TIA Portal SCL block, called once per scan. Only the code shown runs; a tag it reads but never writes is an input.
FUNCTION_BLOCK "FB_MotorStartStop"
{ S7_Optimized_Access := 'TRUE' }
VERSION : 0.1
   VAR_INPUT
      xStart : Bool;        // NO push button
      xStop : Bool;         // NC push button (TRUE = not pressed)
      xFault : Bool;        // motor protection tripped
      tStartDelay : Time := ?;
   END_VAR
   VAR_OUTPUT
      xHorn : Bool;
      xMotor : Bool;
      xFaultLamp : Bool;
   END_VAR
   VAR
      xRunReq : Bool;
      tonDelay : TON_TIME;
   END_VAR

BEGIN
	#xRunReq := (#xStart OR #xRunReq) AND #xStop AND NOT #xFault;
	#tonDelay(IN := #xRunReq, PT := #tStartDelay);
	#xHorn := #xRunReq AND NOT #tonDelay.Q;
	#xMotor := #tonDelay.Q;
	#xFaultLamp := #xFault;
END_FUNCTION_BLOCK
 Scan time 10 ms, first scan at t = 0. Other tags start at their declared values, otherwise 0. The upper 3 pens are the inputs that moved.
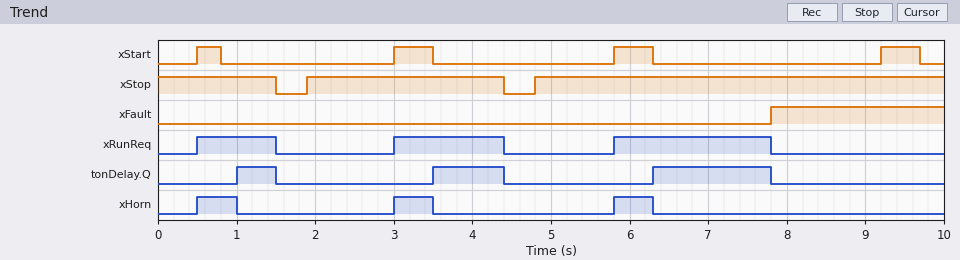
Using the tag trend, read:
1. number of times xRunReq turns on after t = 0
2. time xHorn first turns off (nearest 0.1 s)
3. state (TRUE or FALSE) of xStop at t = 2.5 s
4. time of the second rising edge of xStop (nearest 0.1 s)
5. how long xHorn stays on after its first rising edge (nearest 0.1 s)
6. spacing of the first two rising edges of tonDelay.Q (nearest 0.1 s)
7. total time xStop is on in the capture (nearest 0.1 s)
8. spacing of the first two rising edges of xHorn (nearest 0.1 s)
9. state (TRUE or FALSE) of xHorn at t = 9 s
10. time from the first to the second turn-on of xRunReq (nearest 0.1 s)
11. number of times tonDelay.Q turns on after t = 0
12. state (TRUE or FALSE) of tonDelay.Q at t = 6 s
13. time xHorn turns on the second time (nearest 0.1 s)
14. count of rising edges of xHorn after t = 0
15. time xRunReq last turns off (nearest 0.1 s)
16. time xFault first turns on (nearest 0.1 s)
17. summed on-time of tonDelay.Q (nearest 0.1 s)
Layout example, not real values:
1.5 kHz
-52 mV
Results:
3
1.0 s
TRUE
4.8 s
0.5 s
2.5 s
9.2 s
2.5 s
FALSE
2.5 s
3
FALSE
3.0 s
3
7.8 s
7.8 s
2.9 s
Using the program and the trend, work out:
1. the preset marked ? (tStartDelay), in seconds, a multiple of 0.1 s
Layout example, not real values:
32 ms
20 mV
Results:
0.5 s
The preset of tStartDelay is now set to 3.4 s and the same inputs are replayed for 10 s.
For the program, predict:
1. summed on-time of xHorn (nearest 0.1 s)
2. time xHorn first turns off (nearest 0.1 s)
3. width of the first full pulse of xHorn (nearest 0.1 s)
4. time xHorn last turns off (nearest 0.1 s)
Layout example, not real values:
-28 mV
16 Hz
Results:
4.4 s
1.5 s
1.0 s
7.8 s
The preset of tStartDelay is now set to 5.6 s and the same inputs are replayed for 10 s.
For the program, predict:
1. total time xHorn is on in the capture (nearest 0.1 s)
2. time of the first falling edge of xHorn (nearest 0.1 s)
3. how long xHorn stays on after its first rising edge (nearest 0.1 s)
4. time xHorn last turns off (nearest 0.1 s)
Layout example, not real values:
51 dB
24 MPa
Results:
4.4 s
1.5 s
1.0 s
7.8 s
